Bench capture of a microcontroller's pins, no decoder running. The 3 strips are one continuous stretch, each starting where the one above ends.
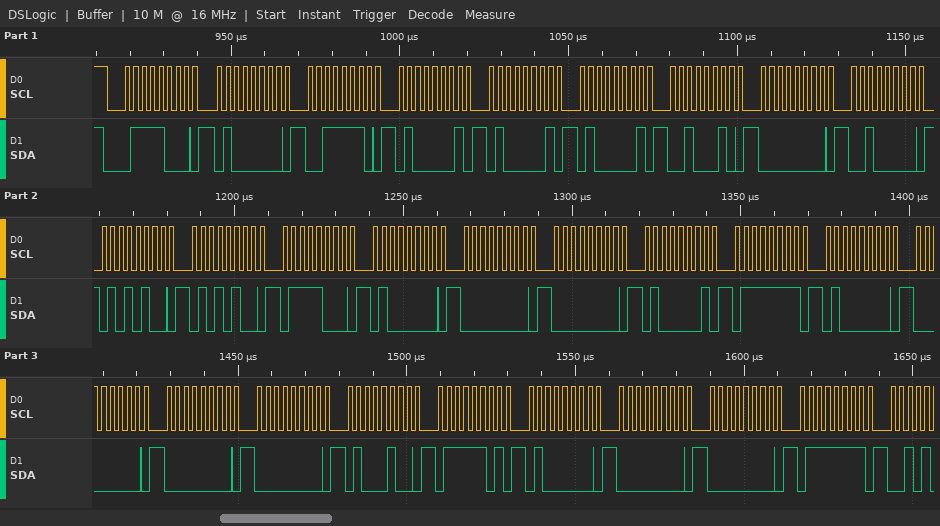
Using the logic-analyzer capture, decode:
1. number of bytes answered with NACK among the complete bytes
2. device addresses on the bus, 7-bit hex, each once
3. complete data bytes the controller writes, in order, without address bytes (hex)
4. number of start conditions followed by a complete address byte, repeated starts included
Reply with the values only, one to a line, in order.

0
0x3C
40 3E 41 41 41 22 00 20 54 54 78 40 00 00 41 7F 40 00 00 00 44 7D 40 00 00 7F
1
